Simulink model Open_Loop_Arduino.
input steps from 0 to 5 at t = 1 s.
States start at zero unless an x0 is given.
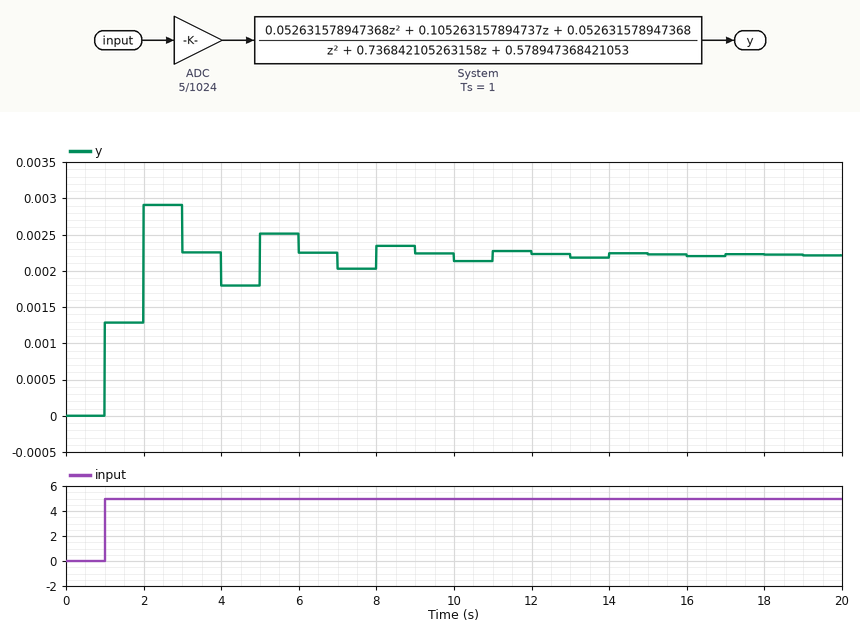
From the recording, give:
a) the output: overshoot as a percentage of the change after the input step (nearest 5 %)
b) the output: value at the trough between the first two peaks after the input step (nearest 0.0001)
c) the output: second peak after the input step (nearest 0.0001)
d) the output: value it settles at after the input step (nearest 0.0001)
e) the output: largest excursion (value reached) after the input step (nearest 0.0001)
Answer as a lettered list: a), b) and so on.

a) 30 %
b) 0.0018
c) 0.0025
d) 0.0022
e) 0.0029
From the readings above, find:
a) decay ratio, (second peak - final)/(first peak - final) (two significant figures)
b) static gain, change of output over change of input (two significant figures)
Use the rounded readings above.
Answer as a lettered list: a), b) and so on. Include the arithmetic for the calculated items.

a) (0.0025 - 0.0022) / (0.0029 - 0.0022) = 0.43
b) (0.0022 - 0) / (5 - 0) = 0.00044
